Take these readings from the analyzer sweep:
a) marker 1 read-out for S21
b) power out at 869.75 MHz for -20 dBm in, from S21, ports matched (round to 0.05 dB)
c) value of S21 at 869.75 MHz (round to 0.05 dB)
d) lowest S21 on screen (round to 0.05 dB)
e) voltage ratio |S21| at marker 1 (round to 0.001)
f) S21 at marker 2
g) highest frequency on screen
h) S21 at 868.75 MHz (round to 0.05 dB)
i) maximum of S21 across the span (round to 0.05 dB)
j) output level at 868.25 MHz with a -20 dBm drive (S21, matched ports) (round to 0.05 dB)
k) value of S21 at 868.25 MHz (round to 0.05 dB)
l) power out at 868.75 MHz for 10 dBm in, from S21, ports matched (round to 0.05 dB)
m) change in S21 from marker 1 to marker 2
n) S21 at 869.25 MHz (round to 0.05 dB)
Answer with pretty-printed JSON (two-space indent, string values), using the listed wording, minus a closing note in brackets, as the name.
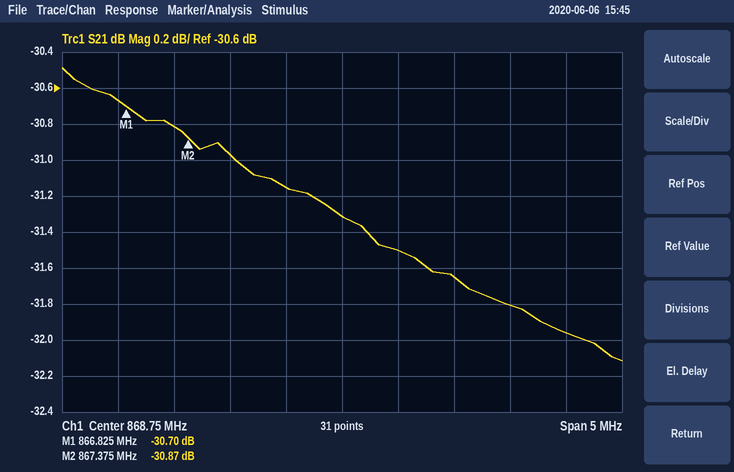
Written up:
{
  "marker 1 read-out for S21": "-30.70 dB",
  "power out at 869.75 MHz for -20 dBm in, from S21, ports matched": "-51.65 dBm",
  "value of S21 at 869.75 MHz": "-31.65 dB",
  "lowest S21 on screen": "-32.10 dB",
  "voltage ratio |S21| at marker 1": "0.029",
  "S21 at marker 2": "-30.87 dB",
  "highest frequency on screen": "871.25 MHz",
  "S21 at 868.75 MHz": "-31.30 dB",
  "maximum of S21 across the span": "-30.50 dB",
  "output level at 868.25 MHz with a -20 dBm drive (S21, matched ports)": "-51.15 dBm",
  "value of S21 at 868.25 MHz": "-31.15 dB",
  "power out at 868.75 MHz for 10 dBm in, from S21, ports matched": "-21.30 dBm",
  "change in S21 from marker 1 to marker 2": "-0.17 dB",
  "S21 at 869.25 MHz": "-31.50 dB"
}
